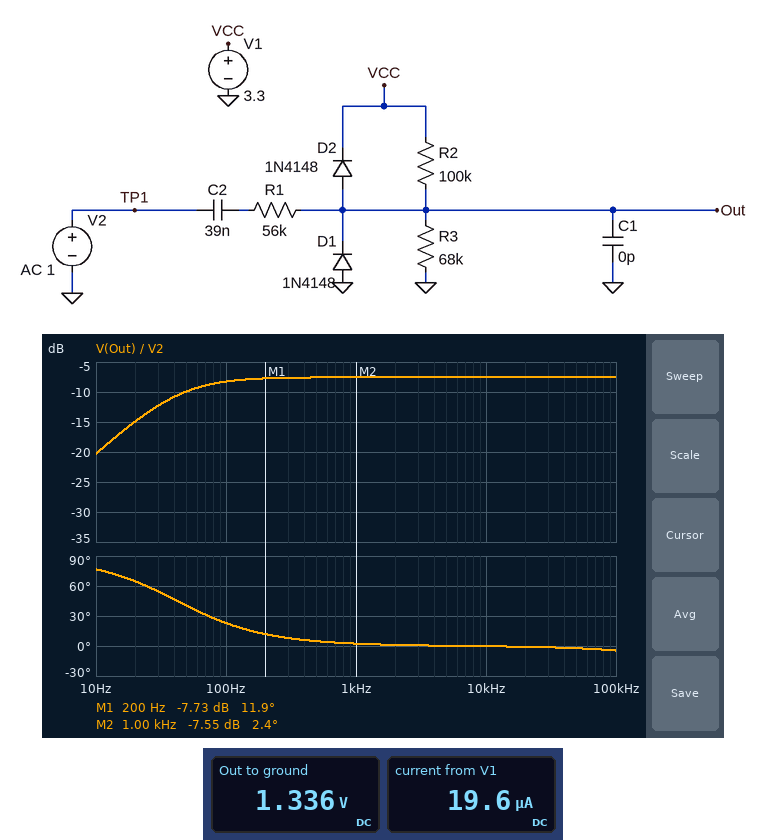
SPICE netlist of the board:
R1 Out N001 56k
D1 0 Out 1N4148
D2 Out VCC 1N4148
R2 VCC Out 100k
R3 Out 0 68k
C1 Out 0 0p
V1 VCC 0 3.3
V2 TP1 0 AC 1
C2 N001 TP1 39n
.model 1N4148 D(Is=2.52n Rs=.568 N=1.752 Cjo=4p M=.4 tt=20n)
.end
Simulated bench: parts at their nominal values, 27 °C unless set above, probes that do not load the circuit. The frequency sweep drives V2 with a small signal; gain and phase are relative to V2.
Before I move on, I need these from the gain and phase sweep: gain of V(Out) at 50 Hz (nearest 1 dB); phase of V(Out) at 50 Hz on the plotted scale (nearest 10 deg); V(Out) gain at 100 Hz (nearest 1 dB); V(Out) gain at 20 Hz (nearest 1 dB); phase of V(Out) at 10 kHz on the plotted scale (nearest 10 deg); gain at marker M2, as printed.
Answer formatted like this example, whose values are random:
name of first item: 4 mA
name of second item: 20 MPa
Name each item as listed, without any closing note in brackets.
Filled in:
gain of V(Out) at 50 Hz: -10 dB
phase of V(Out) at 50 Hz on the plotted scale: 40 deg
V(Out) gain at 100 Hz: -8 dB
V(Out) gain at 20 Hz: -15 dB
phase of V(Out) at 10 kHz on the plotted scale: 0 deg
gain at marker M2, as printed: -7.55 dB
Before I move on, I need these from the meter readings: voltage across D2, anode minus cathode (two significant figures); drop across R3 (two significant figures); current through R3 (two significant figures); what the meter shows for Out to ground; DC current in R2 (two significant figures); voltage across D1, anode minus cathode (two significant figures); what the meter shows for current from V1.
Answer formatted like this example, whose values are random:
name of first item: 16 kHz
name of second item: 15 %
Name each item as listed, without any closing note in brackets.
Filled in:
voltage across D2, anode minus cathode: -2.0 V
drop across R3: 1.3 V
current through R3: 20 µA
what the meter shows for Out to ground: 1.336 V
DC current in R2: 20 µA
voltage across D1, anode minus cathode: -1.3 V
what the meter shows for current from V1: 19.6 µA
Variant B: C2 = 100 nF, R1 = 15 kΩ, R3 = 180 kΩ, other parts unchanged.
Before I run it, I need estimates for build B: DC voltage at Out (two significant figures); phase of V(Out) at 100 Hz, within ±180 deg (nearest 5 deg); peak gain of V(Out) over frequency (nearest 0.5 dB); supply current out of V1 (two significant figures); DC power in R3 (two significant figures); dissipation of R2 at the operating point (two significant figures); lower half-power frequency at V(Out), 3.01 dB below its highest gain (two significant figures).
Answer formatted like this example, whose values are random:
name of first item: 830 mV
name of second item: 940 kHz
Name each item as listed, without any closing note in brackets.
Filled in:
DC voltage at Out: 2.1 V
phase of V(Out) at 100 Hz, within ±180 deg: 10 deg
peak gain of V(Out) over frequency: -2.0 dB
supply current out of V1: 12 µA
DC power in R3: 25 µW
dissipation of R2 at the operating point: 14 µW
lower half-power frequency at V(Out), 3.01 dB below its highest gain: 20 Hz
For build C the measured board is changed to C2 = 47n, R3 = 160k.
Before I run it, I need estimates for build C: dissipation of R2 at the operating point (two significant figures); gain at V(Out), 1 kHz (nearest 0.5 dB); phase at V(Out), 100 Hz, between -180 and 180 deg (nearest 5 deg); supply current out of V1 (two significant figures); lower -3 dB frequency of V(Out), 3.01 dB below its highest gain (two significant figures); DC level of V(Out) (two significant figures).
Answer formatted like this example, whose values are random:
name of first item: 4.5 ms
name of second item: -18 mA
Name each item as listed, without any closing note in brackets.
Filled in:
dissipation of R2 at the operating point: 16 µW
gain at V(Out), 1 kHz: -5.5 dB
phase at V(Out), 100 Hz, between -180 and 180 deg: 15 deg
supply current out of V1: 13 µA
lower -3 dB frequency of V(Out), 3.01 dB below its highest gain: 29 Hz
DC level of V(Out): 2.0 V
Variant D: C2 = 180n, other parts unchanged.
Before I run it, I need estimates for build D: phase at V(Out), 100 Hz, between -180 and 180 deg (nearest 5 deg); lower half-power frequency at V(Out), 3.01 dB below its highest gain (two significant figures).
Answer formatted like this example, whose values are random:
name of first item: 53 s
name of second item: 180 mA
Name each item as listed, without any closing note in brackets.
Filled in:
phase at V(Out), 100 Hz, between -180 and 180 deg: 5 deg
lower half-power frequency at V(Out), 3.01 dB below its highest gain: 9.2 Hz
